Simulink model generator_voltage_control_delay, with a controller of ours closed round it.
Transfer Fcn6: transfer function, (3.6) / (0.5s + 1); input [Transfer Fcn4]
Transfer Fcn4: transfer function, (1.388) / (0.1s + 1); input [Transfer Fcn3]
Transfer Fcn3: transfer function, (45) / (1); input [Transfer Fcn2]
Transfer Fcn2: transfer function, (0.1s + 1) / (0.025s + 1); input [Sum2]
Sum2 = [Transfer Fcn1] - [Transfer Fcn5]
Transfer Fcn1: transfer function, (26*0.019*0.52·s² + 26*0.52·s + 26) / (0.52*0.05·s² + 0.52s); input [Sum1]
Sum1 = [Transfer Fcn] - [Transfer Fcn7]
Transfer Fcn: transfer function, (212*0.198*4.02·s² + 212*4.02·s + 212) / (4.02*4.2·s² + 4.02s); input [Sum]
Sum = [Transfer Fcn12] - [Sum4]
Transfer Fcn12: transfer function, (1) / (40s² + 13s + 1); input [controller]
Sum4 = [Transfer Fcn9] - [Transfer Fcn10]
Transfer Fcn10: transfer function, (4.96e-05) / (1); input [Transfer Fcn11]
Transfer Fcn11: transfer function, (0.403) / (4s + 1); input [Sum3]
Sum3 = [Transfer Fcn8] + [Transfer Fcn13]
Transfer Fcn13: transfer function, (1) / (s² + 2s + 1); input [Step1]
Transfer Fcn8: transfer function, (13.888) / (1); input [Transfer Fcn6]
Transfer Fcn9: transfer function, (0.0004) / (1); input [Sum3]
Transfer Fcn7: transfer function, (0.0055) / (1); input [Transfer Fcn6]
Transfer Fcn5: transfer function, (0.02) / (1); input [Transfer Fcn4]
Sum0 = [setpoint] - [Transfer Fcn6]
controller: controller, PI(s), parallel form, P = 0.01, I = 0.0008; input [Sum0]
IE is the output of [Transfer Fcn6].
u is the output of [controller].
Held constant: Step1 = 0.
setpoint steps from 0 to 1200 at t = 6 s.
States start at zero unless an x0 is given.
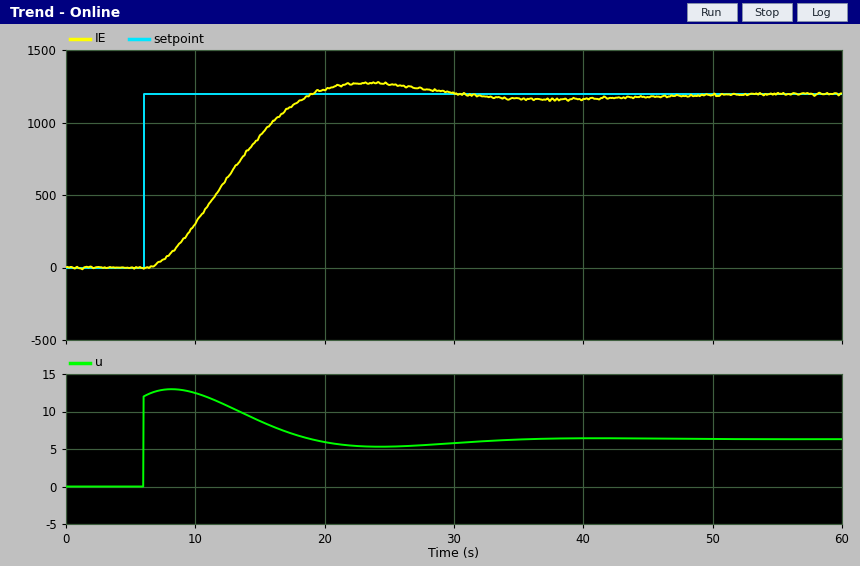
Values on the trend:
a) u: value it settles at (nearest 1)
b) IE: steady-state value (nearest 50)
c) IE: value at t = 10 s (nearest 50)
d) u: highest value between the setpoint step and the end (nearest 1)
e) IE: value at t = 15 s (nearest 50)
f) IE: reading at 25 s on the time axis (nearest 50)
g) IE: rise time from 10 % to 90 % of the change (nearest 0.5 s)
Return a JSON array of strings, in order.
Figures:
["6", "1200", "300", "13", "900", "1250", "8.5 s"]
